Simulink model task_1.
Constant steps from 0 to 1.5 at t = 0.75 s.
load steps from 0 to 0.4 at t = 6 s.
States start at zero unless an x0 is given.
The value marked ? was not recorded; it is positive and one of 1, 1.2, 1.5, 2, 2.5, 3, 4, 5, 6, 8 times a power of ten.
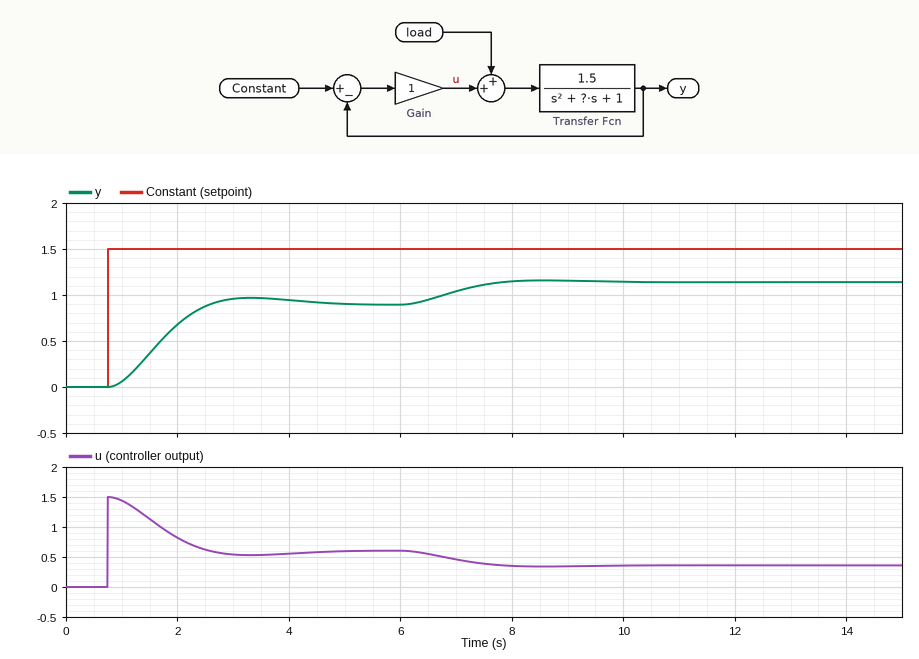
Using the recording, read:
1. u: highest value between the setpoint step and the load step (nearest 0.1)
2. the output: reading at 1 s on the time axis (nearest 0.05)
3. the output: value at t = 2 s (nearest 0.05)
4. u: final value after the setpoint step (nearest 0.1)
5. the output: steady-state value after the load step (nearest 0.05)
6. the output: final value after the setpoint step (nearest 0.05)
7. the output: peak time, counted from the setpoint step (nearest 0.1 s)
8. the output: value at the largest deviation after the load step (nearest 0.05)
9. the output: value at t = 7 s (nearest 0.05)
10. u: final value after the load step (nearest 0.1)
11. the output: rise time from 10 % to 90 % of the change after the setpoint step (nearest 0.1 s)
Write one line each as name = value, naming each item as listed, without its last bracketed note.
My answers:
u: highest value between the setpoint step and the load step = 1.5
the output: reading at 1 s on the time axis = 0.05
the output: value at t = 2 s = 0.70
u: final value after the setpoint step = 0.6
the output: steady-state value after the load step = 1.15
the output: final value after the setpoint step = 0.90
the output: peak time, counted from the setpoint step = 2.6 s
the output: value at the largest deviation after the load step = 1.15
the output: value at t = 7 s = 1.05
u: final value after the load step = 0.4
the output: rise time from 10 % to 90 % of the change after the setpoint step = 1.2 s
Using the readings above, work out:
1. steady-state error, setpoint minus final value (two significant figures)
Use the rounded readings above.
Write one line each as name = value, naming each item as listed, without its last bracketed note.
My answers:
steady-state error, setpoint minus final value = 0.60
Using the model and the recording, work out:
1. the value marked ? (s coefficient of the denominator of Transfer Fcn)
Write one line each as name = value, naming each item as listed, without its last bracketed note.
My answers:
the value marked ? = 2
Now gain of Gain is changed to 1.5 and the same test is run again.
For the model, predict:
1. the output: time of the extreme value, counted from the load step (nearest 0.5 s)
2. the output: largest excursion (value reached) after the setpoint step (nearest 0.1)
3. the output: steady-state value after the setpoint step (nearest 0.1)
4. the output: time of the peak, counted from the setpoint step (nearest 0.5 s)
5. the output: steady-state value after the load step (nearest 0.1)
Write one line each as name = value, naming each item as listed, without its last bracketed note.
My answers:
the output: time of the extreme value, counted from the load step = 2.0 s
the output: largest excursion (value reached) after the setpoint step = 1.2
the output: steady-state value after the setpoint step = 1.0
the output: time of the peak, counted from the setpoint step = 2.0 s
the output: steady-state value after the load step = 1.2
